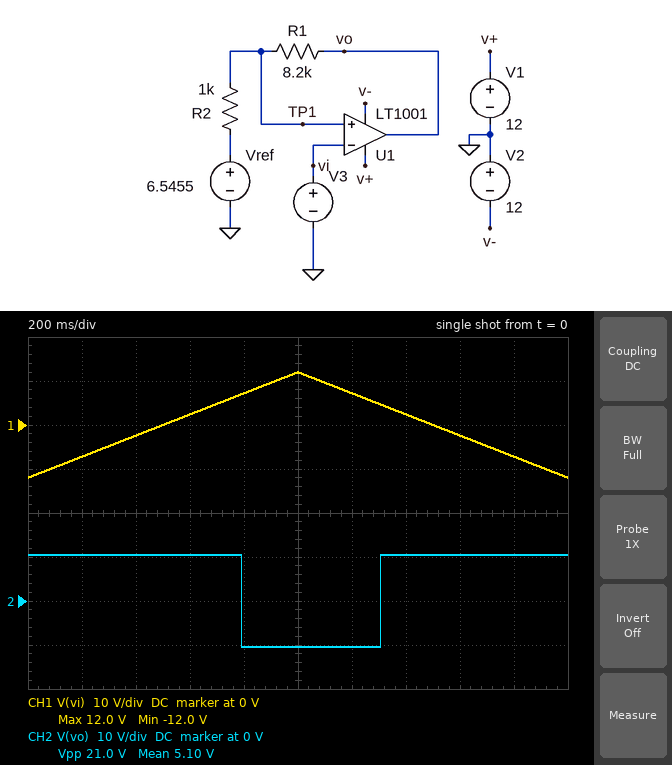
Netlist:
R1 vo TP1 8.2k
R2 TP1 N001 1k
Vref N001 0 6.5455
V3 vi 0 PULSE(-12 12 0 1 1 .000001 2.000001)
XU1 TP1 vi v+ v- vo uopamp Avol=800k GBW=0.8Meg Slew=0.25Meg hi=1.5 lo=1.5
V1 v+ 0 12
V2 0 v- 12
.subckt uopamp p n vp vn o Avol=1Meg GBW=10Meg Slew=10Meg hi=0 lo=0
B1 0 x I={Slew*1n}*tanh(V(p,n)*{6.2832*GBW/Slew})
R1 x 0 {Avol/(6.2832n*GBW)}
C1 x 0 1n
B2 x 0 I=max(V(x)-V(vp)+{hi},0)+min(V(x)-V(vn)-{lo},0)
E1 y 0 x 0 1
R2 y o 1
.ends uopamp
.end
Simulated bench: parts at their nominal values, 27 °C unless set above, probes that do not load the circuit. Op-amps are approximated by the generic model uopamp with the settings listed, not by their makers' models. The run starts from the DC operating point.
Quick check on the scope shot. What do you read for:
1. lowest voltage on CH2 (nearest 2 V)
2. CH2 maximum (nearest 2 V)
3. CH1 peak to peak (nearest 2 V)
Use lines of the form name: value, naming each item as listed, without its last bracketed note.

lowest voltage on CH2: -10 V
CH2 maximum: 10 V
CH1 peak to peak: 24 V
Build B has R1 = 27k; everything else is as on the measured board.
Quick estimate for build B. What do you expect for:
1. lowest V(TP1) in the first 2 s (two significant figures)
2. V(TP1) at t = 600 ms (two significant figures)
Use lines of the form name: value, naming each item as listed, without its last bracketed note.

lowest V(TP1) in the first 2 s: 5.9 V
V(TP1) at t = 600 ms: 6.7 V
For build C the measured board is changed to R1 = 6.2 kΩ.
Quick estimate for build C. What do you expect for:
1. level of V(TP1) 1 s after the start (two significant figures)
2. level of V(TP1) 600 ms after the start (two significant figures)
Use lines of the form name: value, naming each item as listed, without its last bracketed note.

level of V(TP1) 1 s after the start: 4.2 V
level of V(TP1) 600 ms after the start: 7.1 V
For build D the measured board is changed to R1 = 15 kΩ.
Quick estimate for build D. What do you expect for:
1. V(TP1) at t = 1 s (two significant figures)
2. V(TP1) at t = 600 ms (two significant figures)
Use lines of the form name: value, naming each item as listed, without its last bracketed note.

V(TP1) at t = 1 s: 5.5 V
V(TP1) at t = 600 ms: 6.8 V
